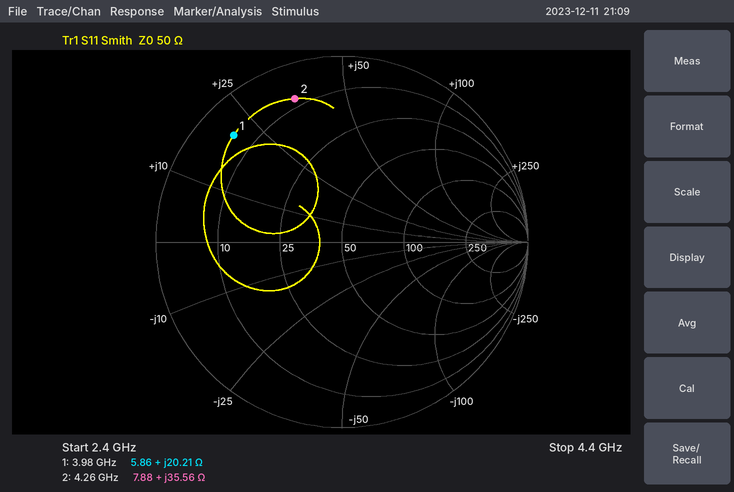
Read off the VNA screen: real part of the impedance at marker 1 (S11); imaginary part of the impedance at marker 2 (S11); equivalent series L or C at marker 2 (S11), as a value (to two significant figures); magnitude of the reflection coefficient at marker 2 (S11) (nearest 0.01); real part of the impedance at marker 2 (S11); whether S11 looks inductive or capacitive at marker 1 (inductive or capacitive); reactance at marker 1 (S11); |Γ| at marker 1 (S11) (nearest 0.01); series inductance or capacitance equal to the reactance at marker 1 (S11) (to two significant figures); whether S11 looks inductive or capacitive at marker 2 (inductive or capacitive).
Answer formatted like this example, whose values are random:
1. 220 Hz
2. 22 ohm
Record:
1. 5.86 Ω
2. +35.56 Ω
3. 1.3 nH
4. 0.81
5. 7.88 Ω
6. inductive
7. +20.21 Ω
8. 0.82
9. 810 pH
10. inductive
